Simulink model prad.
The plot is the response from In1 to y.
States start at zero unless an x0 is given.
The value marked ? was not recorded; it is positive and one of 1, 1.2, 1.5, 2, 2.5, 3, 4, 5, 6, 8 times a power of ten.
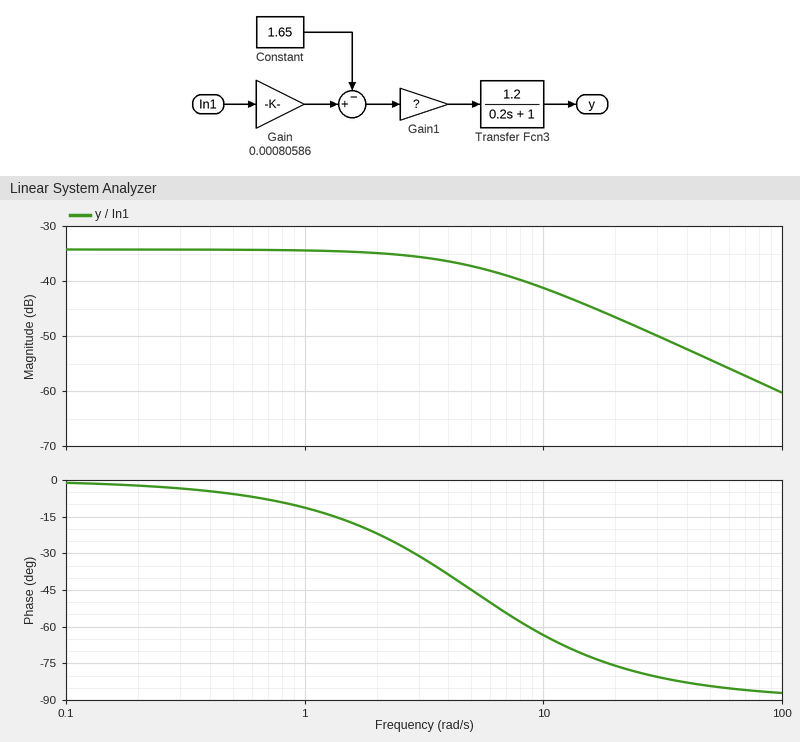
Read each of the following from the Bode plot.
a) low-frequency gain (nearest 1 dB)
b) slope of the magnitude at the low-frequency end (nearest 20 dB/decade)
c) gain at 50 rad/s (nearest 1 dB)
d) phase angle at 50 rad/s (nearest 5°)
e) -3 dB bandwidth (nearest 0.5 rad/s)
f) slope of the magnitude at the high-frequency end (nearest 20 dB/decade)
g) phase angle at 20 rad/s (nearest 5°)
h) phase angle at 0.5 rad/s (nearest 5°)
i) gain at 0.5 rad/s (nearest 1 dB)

-34 dB
0 dB/decade
-54 dB
-85°
5.0 rad/s
-20 dB/decade
-75°
-5°
-34 dB
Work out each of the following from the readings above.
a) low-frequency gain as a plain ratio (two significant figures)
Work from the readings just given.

0.020
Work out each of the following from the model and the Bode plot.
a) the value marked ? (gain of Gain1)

20
